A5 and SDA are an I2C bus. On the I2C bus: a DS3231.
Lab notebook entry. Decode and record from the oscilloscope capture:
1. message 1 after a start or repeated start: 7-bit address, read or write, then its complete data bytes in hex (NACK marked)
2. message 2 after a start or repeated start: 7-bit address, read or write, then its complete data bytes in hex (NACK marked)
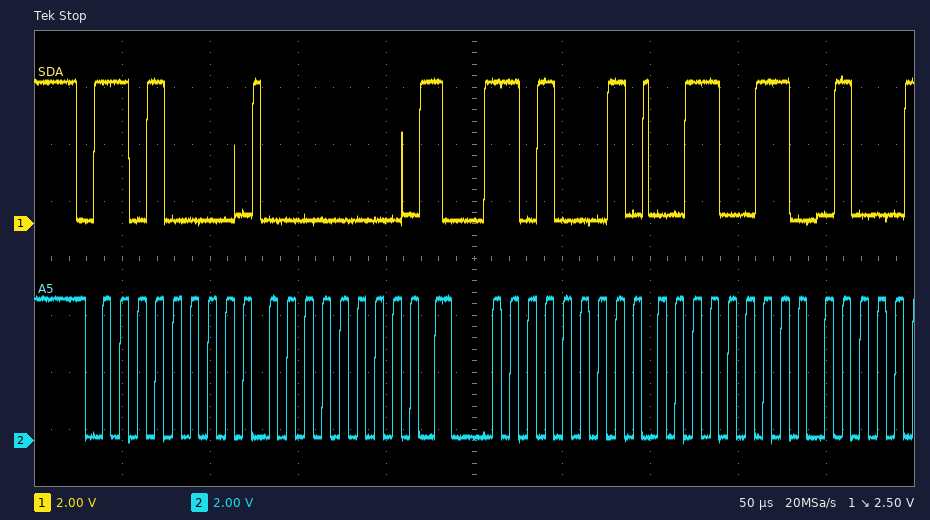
0x68 write: 00
0x68 read: 33
